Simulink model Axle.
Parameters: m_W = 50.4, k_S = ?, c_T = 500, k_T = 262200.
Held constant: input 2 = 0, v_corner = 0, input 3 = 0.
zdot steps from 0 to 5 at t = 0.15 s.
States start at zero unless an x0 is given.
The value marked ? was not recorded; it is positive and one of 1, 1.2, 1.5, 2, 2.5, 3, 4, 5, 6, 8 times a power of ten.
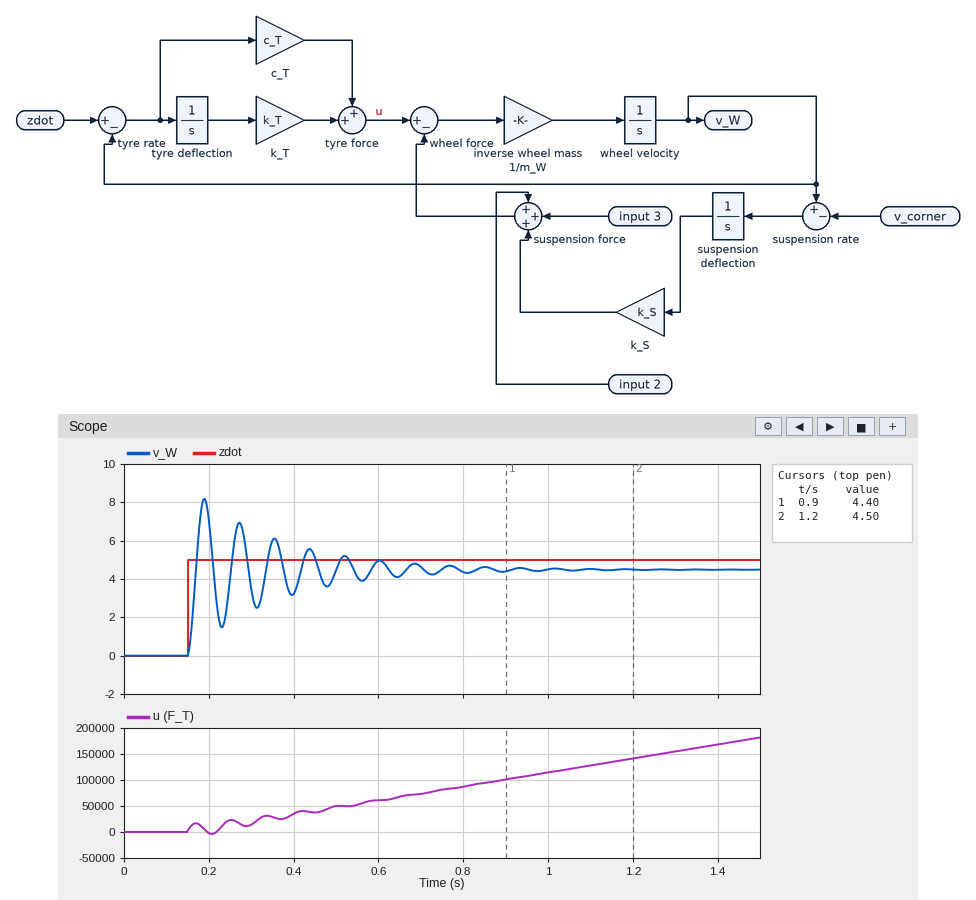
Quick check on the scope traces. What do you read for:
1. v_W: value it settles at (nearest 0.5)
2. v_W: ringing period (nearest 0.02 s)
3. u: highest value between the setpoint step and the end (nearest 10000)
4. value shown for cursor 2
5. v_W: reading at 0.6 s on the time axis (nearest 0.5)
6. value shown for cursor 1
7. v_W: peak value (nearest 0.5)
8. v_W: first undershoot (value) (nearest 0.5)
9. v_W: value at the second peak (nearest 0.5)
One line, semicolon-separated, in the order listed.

4.5; 0.08 s; 180000; 4.50; 5.0; 4.40; 8.0; 1.5; 7.0
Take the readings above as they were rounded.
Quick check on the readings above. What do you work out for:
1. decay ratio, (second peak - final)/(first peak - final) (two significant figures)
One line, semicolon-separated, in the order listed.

0.71
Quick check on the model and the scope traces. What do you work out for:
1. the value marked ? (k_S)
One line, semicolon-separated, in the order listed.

30000
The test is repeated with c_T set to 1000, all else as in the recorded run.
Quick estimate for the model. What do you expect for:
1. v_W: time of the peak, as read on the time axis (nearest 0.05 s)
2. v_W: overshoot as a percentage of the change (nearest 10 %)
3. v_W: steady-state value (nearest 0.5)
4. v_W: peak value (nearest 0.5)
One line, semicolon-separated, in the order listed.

0.20 s; 70 %; 4.5; 7.5
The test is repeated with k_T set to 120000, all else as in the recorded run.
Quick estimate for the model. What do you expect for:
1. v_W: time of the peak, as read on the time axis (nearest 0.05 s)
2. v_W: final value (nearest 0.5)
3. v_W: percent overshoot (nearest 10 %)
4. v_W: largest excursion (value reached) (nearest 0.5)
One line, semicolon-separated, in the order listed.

0.20 s; 4.0; 80 %; 7.0
